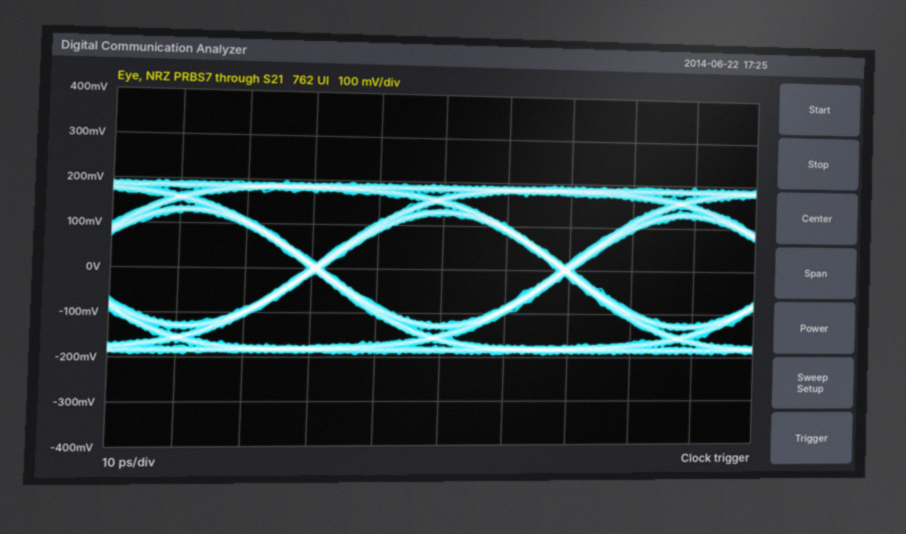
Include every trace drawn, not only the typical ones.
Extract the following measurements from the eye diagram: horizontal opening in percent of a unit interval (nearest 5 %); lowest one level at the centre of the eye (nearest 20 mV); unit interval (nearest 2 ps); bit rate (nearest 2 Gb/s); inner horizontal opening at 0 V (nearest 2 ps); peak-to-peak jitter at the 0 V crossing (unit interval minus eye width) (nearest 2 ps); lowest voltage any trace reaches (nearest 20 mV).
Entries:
95 %
120 mV
38 ps
26 Gb/s
36 ps
2 ps
-200 mV
